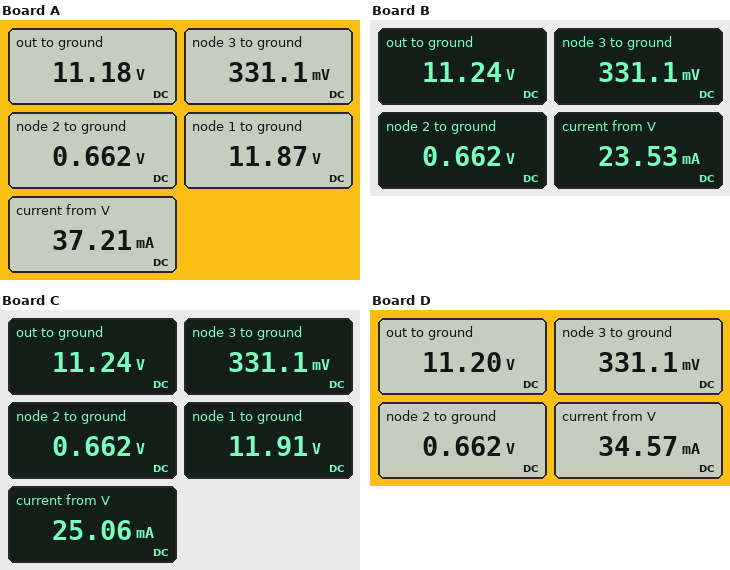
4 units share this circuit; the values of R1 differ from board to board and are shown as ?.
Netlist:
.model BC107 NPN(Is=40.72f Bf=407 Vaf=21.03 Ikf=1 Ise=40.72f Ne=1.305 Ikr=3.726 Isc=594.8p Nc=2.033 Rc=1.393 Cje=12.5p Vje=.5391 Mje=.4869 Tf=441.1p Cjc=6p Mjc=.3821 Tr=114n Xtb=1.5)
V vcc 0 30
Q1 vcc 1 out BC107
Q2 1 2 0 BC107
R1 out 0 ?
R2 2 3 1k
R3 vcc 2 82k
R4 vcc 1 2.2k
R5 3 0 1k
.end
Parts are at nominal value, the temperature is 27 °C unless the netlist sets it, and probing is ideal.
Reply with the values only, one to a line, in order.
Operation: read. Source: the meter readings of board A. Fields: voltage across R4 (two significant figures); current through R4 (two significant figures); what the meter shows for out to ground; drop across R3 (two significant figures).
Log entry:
18 V
8.2 mA
11.18 V
29 V
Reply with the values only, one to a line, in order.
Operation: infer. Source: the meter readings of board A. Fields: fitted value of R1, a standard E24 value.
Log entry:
390 Ω
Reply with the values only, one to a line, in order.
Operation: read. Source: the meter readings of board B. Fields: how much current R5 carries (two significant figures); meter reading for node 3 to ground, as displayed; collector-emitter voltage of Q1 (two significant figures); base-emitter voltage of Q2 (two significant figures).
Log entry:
330 µA
331.1 mV
19 V
660 mV
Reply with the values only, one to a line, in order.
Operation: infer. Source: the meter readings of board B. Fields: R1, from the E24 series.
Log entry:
750 Ω
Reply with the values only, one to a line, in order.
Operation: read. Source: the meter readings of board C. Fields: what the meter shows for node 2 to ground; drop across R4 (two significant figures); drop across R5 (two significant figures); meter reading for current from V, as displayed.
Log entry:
0.662 V
18 V
330 mV
25.06 mA
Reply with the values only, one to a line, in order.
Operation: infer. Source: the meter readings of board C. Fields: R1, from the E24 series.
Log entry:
680 Ω
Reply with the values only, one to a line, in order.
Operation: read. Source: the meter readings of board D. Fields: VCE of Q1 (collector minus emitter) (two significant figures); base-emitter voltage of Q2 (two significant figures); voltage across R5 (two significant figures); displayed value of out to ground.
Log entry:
19 V
660 mV
330 mV
11.20 V
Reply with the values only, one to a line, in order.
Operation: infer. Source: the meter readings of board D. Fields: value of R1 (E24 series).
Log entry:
430 Ω
